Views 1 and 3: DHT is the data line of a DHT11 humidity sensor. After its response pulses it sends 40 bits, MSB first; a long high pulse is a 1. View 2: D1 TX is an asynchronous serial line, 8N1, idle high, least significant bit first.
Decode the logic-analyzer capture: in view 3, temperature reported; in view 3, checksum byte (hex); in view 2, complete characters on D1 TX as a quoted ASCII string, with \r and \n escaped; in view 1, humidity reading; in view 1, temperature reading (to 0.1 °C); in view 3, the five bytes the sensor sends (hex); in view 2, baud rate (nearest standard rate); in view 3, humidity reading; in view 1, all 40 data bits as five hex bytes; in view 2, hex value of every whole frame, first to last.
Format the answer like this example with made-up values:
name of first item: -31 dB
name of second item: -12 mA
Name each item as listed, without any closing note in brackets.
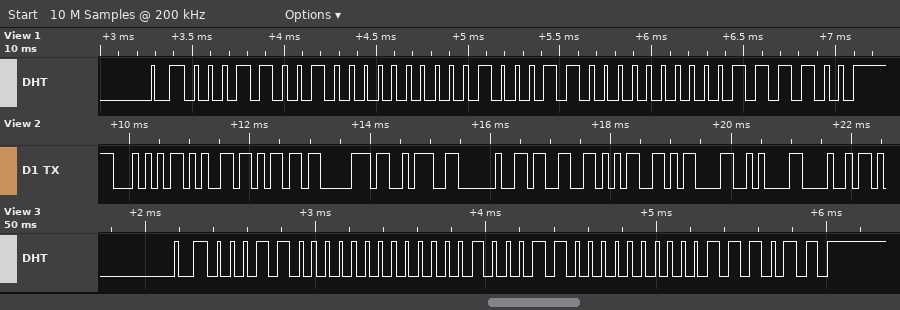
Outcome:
in view 3, temperature reported: 35.0 °C
in view 3, checksum byte: 0x3B
in view 2, complete characters on D1 TX as a quoted ASCII string, with \r and \n escaped: "Temp: 35\r\nH"
in view 1, humidity reading: 25 %
in view 1, temperature reading: 35.0 °C
in view 3, the five bytes the sensor sends: 18 00 23 00 3B
in view 2, baud rate: 9600 baud
in view 3, humidity reading: 24 %
in view 1, all 40 data bits as five hex bytes: 19 00 23 00 3C
in view 2, hex value of every whole frame, first to last: 54 65 6D 70 3A 20 33 35 0D 0A 48
